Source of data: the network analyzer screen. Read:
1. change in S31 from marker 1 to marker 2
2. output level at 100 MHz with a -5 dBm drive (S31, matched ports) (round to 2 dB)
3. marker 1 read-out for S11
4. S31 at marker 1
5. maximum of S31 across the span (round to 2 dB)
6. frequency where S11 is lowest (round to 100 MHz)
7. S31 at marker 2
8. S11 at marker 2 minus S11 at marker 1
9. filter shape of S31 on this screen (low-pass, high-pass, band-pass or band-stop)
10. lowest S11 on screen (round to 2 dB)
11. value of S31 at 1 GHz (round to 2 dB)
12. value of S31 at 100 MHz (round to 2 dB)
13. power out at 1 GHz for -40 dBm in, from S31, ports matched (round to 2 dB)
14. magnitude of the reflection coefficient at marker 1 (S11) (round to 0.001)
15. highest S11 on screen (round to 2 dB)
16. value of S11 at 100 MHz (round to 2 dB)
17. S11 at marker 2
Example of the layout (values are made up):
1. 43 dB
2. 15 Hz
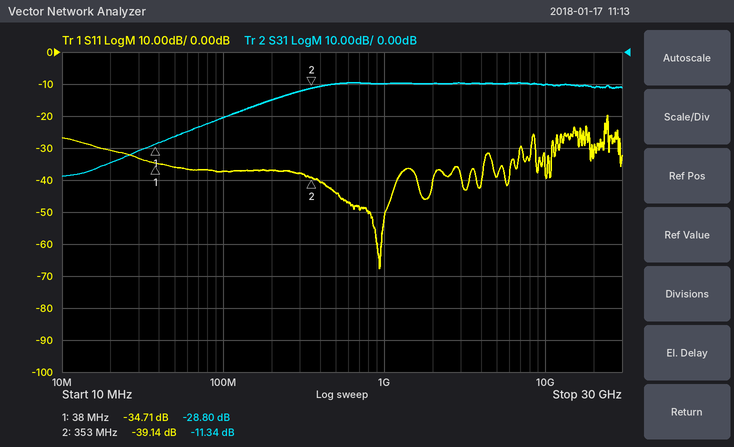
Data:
1. 17.46 dB
2. -26 dBm
3. -34.71 dB
4. -28.80 dB
5. -10 dB
6. 900 MHz
7. -11.34 dB
8. -4.43 dB
9. high-pass
10. -68 dB
11. -10 dB
12. -20 dB
13. -50 dBm
14. 0.018
15. -20 dB
16. -38 dB
17. -39.14 dB
